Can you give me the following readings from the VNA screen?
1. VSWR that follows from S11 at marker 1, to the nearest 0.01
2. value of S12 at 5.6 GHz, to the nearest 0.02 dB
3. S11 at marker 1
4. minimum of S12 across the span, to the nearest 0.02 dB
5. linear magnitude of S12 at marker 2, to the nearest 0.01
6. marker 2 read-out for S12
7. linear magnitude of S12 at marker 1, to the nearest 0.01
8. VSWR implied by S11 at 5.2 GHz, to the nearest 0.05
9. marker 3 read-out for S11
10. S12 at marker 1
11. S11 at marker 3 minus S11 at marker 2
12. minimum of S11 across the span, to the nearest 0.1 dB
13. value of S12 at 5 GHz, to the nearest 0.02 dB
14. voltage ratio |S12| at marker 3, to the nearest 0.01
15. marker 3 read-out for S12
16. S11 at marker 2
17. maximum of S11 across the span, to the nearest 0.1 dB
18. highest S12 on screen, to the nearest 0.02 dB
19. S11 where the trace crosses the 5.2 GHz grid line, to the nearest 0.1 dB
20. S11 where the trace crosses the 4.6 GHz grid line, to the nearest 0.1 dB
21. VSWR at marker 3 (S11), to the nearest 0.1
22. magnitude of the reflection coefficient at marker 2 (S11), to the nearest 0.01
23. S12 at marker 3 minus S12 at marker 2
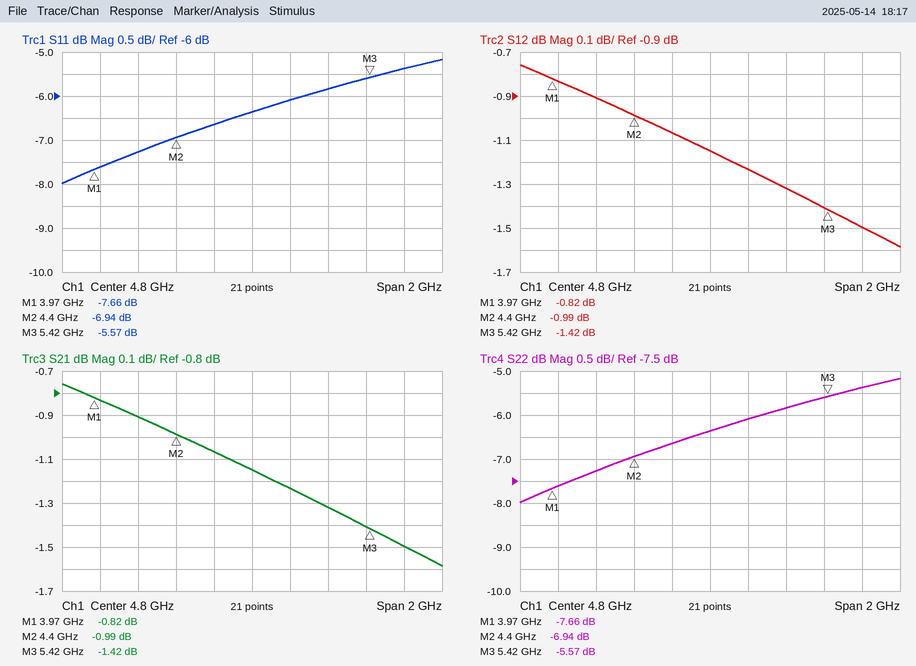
2.41
-1.50 dB
-7.66 dB
-1.58 dB
0.89
-0.99 dB
0.91
3.10
-5.57 dB
-0.82 dB
1.37 dB
-8.0 dB
-1.24 dB
0.85
-1.42 dB
-6.94 dB
-5.2 dB
-0.76 dB
-5.8 dB
-6.6 dB
3.2
0.45
-0.43 dB
